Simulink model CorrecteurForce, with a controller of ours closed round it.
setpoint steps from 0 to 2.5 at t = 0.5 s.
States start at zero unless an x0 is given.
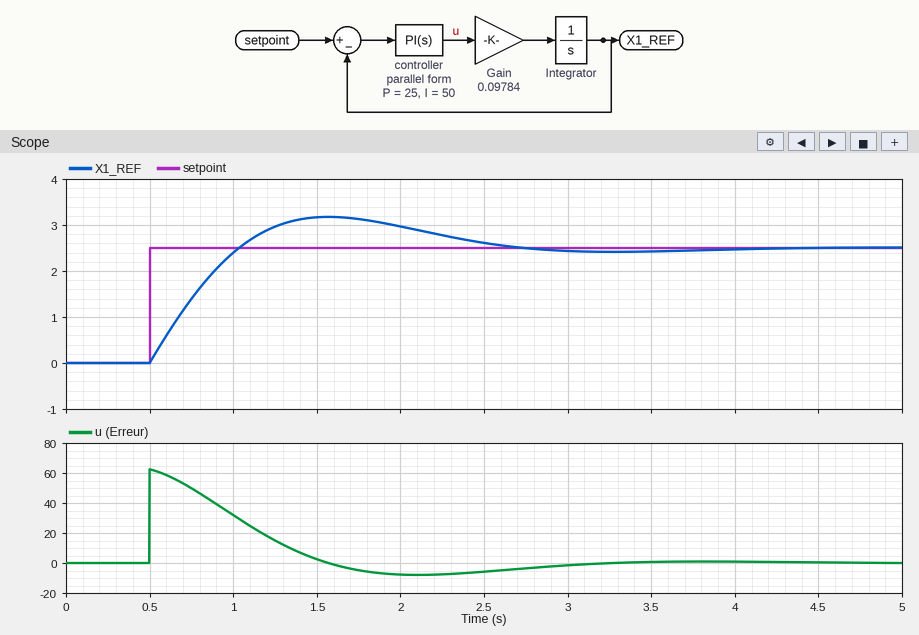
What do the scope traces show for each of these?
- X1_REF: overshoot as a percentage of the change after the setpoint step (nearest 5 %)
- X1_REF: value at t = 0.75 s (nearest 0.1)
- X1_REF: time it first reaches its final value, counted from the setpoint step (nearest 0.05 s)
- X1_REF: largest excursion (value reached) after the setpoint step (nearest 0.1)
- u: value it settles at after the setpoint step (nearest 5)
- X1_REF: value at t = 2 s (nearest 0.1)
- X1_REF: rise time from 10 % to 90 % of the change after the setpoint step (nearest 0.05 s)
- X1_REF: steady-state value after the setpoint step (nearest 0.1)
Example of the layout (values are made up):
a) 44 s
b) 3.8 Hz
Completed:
a) 25 %
b) 1.4
c) 0.55 s
d) 3.2
e) 0
f) 3.0
g) 0.40 s
h) 2.5
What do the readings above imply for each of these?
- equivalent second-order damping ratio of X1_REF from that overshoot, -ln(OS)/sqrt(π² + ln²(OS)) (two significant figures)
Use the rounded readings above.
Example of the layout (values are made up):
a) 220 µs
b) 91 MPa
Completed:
a) 0.40
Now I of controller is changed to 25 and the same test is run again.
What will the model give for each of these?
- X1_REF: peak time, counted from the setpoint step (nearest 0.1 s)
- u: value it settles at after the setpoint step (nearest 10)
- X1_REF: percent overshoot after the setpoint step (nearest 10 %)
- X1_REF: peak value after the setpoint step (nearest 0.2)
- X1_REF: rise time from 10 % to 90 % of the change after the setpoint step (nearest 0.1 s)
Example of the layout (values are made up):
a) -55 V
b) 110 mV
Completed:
a) 1.4 s
b) 0
c) 20 %
d) 3.0
e) 0.5 s
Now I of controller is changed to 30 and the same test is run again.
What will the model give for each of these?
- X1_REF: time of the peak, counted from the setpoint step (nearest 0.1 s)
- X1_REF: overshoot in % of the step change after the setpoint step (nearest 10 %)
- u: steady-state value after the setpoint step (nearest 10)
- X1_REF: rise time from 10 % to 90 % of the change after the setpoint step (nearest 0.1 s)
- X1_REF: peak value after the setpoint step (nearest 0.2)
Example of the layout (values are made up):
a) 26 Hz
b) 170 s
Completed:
a) 1.3 s
b) 20 %
c) 0
d) 0.5 s
e) 3.0
